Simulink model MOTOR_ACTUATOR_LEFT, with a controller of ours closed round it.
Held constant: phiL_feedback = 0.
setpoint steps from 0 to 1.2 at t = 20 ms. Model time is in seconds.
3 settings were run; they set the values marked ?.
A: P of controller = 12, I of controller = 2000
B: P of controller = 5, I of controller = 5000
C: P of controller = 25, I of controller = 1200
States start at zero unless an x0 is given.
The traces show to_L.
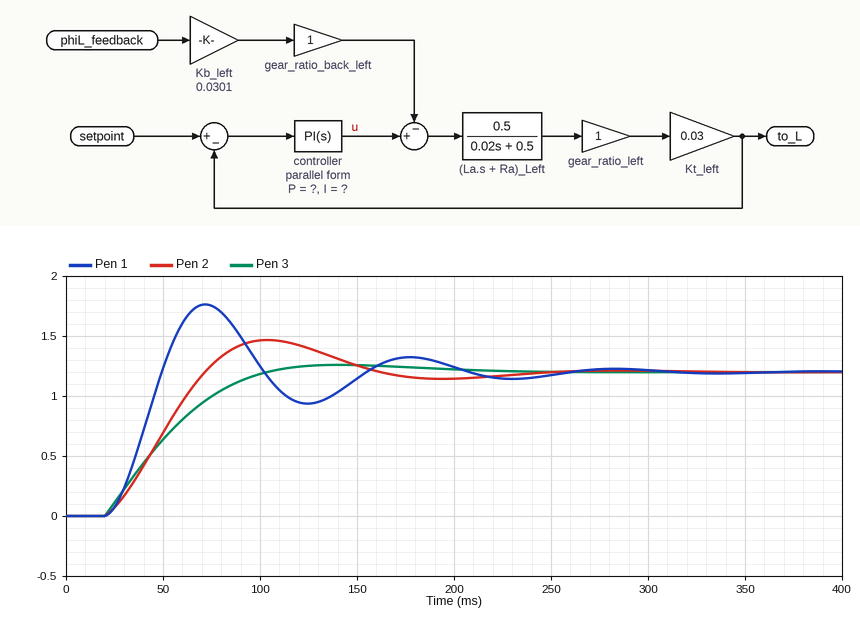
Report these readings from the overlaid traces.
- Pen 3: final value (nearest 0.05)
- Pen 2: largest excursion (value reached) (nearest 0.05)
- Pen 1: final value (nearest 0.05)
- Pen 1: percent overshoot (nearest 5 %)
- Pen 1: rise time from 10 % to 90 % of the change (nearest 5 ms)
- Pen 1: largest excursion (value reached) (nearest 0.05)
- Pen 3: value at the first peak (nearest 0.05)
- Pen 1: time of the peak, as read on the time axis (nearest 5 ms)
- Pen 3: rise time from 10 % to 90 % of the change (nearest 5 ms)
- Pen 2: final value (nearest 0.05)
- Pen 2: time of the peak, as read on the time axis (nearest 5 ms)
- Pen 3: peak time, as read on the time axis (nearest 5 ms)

1.20
1.45
1.20
45 %
20 ms
1.75
1.25
70 ms
60 ms
1.20
105 ms
140 ms
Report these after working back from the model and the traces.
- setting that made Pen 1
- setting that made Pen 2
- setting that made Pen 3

B
A
C
